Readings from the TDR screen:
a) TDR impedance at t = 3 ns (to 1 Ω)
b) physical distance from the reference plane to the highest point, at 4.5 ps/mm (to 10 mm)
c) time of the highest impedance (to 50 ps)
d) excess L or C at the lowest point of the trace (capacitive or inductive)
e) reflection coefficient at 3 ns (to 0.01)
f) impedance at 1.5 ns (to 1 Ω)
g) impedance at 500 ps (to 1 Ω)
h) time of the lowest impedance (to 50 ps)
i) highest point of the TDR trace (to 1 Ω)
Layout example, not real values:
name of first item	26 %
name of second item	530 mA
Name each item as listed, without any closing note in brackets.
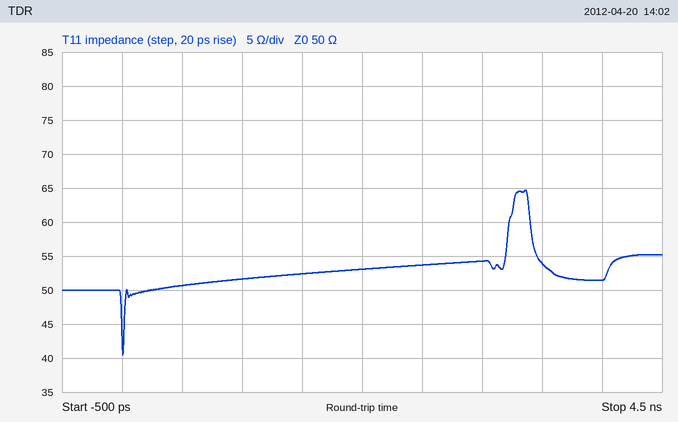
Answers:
TDR impedance at t = 3 ns	54 Ω
physical distance from the reference plane to the highest point, at 4.5 ps/mm	370 mm
time of the highest impedance	3.35 ns
excess L or C at the lowest point of the trace	capacitive
reflection coefficient at 3 ns	+0.04
impedance at 1.5 ns	52 Ω
impedance at 500 ps	51 Ω
time of the lowest impedance	0 ps
highest point of the TDR trace	65 Ω
